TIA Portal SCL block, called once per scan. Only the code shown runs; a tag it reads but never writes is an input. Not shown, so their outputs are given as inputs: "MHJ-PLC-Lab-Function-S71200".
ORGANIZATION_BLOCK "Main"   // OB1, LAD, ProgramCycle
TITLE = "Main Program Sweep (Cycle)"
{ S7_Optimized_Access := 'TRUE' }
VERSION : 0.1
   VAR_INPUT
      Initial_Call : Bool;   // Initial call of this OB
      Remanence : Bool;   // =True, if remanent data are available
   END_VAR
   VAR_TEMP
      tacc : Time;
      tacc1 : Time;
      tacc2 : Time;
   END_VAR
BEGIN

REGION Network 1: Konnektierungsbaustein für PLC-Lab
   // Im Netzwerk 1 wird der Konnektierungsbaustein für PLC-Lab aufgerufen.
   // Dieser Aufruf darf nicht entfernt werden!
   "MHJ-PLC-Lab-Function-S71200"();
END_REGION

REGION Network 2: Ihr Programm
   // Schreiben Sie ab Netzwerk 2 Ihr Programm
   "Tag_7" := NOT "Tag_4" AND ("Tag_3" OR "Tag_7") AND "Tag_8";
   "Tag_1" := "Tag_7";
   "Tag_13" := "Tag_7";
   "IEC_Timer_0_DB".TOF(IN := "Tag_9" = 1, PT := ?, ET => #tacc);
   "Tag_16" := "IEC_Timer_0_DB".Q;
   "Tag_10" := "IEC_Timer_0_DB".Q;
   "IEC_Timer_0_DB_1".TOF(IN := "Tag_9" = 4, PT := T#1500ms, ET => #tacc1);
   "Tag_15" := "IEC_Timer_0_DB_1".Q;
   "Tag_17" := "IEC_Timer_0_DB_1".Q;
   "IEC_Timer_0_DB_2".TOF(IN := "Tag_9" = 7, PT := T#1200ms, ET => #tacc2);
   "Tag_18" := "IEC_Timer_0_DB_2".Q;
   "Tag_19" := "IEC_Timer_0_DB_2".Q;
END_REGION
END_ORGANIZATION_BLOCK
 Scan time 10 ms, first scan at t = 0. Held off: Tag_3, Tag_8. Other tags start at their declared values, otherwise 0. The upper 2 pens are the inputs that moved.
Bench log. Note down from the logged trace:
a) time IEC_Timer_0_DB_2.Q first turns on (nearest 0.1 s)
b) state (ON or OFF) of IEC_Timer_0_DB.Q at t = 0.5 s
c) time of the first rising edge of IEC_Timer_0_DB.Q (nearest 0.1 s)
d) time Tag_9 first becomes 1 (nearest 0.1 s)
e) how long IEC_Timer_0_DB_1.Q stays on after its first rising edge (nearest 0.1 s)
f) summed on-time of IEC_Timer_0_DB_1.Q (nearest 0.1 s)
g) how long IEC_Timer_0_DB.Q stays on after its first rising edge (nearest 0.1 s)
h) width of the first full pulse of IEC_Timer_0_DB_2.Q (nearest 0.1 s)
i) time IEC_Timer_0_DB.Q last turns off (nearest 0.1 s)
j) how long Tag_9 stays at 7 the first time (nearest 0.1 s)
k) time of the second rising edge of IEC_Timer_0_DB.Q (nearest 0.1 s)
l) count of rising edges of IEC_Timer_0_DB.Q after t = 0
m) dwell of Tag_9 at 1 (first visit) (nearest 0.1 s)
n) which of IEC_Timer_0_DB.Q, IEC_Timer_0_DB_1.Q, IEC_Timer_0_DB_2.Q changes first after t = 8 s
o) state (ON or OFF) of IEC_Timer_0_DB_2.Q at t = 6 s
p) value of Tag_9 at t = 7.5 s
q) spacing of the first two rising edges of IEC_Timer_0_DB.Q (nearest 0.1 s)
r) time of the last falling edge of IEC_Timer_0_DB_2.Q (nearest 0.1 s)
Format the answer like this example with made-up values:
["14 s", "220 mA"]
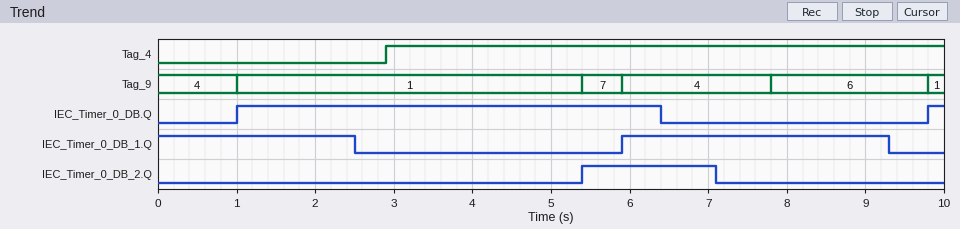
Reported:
["5.4 s", "OFF", "1.0 s", "1.0 s", "3.4 s", "5.9 s", "5.4 s", "1.7 s", "6.4 s", "0.5 s", "9.8 s", "2", "4.4 s", "IEC_Timer_0_DB_1.Q", "ON", "4", "8.8 s", "7.1 s"]
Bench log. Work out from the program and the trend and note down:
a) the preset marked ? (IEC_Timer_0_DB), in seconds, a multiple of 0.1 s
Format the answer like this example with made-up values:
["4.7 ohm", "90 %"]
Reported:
["1.0 s"]
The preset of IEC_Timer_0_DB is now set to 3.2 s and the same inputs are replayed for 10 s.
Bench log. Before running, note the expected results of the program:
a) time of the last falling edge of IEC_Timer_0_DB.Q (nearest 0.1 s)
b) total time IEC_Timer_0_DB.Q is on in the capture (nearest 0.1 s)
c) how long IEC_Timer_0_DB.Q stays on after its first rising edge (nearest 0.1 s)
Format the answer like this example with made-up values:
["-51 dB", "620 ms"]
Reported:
["8.6 s", "7.8 s", "7.6 s"]
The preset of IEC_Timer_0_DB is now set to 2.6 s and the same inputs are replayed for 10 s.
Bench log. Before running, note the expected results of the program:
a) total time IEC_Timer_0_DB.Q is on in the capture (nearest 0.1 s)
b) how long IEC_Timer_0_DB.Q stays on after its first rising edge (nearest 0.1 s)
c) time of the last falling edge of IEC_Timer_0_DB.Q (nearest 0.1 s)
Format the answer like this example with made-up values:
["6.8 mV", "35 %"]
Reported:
["7.2 s", "7.0 s", "8.0 s"]
